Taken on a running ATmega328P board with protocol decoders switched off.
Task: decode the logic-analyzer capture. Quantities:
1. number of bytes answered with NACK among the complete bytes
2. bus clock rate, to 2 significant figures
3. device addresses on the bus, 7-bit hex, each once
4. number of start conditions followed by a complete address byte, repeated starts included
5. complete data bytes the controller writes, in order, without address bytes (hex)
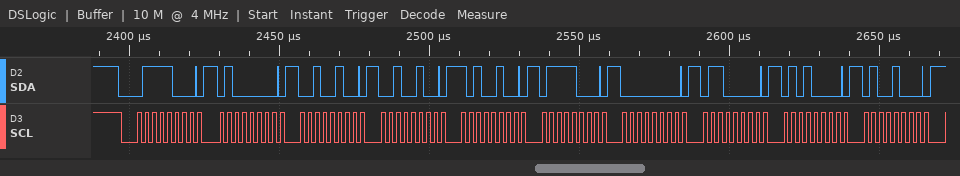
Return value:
0
400 kHz
0x3C
1
40 24 24 A4 78 00 60 50 48
